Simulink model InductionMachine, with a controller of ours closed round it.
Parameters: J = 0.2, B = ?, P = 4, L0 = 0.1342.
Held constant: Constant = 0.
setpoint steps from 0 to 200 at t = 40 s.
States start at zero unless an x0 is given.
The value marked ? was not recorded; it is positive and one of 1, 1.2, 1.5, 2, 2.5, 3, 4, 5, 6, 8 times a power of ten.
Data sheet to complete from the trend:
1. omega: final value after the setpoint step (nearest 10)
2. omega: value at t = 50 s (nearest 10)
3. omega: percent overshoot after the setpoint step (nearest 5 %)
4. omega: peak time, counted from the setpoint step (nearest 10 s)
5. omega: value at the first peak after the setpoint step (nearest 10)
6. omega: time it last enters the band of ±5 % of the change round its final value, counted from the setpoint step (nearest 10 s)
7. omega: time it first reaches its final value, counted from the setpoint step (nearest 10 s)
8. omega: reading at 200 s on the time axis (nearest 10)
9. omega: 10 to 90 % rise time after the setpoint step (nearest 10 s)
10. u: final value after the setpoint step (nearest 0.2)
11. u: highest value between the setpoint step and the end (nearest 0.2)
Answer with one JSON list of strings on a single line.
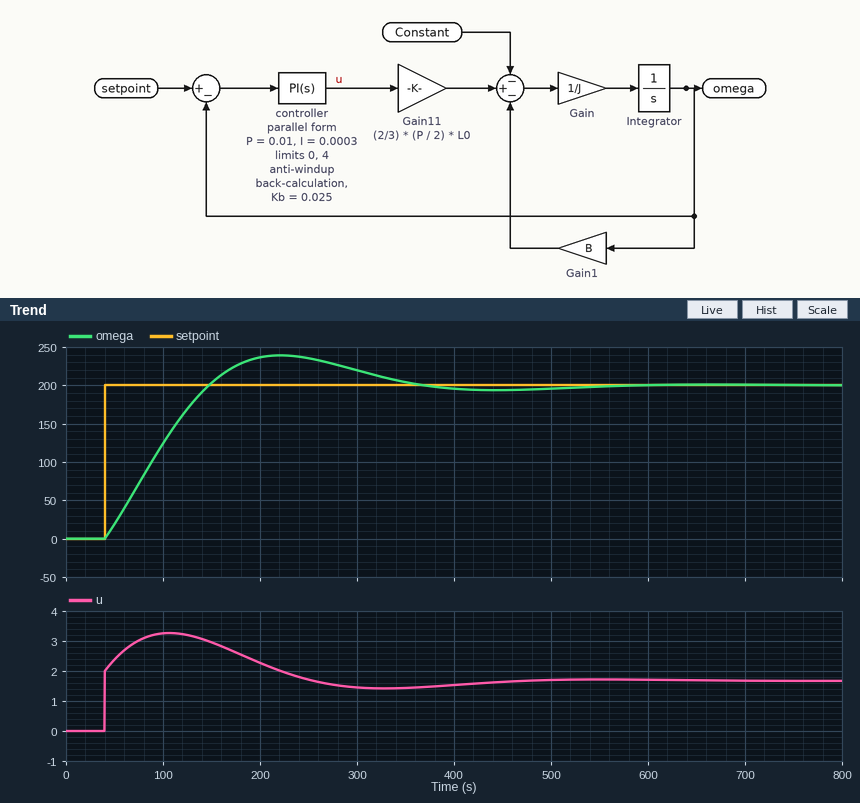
["200", "20", "20 %", "180 s", "240", "290 s", "110 s", "240", "80 s", "1.6", "3.2"]
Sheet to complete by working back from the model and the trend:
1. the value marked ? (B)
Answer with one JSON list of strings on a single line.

["0.0015"]
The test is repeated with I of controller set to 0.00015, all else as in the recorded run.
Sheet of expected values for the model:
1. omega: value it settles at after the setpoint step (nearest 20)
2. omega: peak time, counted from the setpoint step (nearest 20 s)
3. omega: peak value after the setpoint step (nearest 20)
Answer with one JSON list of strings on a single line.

["200", "280 s", "220"]
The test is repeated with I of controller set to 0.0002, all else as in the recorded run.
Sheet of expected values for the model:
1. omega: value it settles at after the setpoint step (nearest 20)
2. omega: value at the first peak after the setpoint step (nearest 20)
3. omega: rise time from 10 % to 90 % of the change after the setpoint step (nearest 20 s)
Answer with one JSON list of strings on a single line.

["200", "220", "100 s"]
